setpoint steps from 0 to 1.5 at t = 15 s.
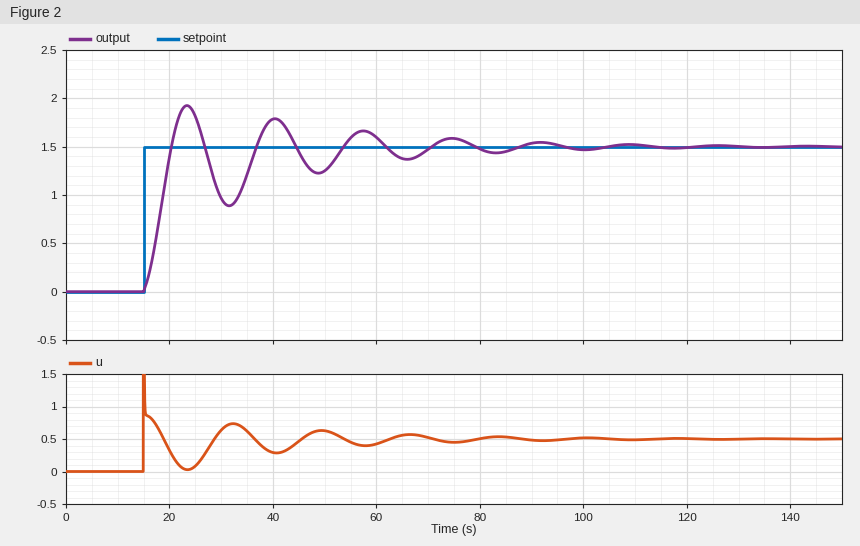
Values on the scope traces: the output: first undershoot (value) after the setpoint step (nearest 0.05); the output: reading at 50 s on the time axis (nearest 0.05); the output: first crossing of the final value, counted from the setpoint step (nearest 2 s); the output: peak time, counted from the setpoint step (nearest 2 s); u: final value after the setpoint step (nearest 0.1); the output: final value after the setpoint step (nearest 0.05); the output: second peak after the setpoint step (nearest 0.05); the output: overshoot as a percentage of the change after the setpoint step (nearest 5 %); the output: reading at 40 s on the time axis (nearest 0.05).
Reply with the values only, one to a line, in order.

0.90
1.25
6 s
8 s
0.5
1.50
1.80
30 %
1.80
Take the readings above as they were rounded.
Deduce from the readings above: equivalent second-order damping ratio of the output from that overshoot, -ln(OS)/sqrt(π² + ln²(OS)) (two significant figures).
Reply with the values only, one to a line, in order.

0.36
